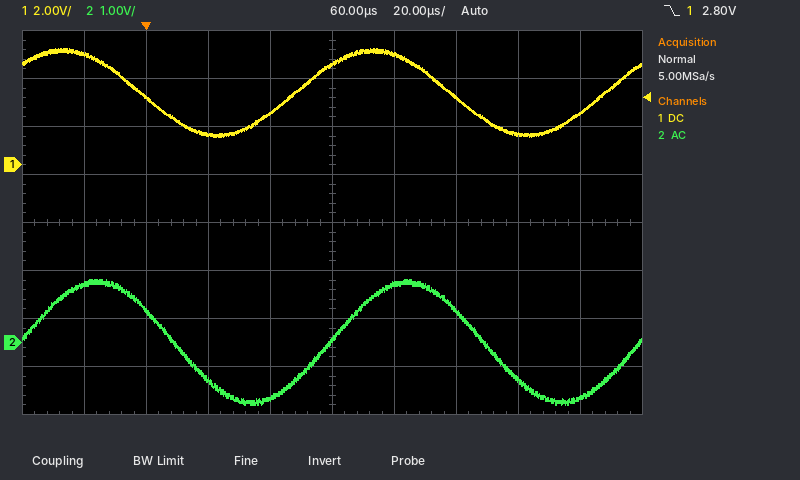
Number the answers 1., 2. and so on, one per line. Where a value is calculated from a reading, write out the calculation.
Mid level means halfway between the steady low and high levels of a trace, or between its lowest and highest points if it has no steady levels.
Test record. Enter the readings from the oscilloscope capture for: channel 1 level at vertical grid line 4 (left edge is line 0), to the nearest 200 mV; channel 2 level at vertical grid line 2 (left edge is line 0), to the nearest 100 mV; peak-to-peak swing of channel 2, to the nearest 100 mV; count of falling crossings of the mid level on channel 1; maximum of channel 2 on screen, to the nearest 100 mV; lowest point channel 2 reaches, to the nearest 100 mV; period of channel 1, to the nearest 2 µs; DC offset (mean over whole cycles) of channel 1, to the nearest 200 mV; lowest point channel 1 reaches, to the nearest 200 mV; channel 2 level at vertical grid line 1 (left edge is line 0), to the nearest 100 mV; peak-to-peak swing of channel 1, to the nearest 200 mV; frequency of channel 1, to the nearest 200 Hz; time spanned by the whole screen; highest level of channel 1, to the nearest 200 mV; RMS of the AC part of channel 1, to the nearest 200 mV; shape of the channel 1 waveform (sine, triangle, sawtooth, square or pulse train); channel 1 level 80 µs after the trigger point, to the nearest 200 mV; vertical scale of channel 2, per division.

1. 2.2 V
2. 700 mV
3. 1.3 V − (-1.3 V) = 2.6 V
4. 2
5. 1.3 V
6. -1.3 V
7. 100 µs
8. (4.8 V + (1.2 V)) / 2 ≈ 3.0 V
9. 1.2 V
10. 1.2 V
11. 4.8 V − (1.2 V) = 3.6 V
12. 1 / 100 µs ≈ 10.0 kHz
13. 200 µs
14. 4.8 V
15. 3.6 V / (2√2) ≈ 1.27 V, so 1.2 V to the nearest 200 mV
16. sine
17. 4.6 V
18. 1 V
